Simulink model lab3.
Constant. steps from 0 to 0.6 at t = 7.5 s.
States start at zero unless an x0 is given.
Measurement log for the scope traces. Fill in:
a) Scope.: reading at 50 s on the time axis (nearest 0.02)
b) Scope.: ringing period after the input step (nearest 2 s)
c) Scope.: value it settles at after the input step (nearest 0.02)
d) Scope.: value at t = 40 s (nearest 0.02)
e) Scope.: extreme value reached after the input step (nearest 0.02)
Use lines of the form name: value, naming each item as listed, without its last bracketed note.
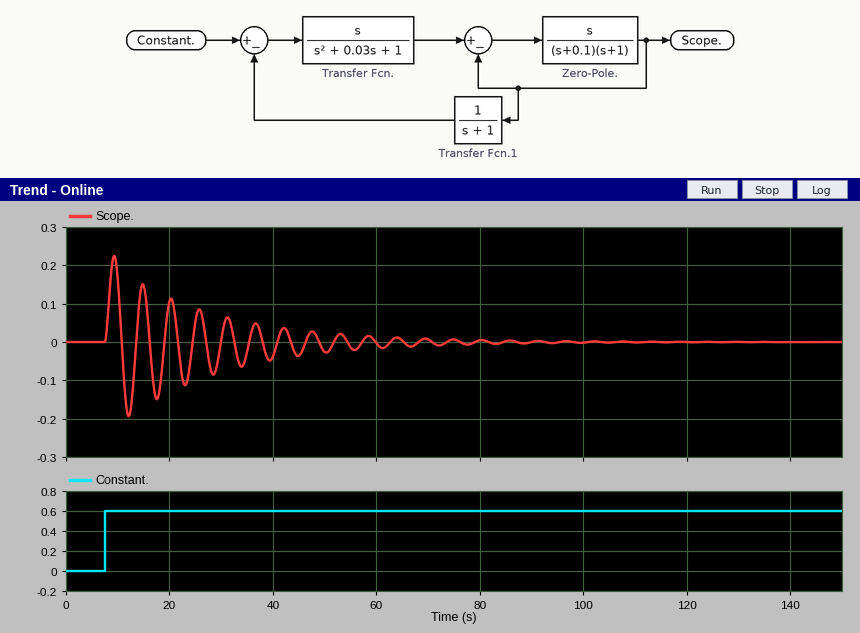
Scope.: reading at 50 s on the time axis: -0.02
Scope.: ringing period after the input step: 6 s
Scope.: value it settles at after the input step: 0.00
Scope.: value at t = 40 s: -0.04
Scope.: extreme value reached after the input step: 0.22
